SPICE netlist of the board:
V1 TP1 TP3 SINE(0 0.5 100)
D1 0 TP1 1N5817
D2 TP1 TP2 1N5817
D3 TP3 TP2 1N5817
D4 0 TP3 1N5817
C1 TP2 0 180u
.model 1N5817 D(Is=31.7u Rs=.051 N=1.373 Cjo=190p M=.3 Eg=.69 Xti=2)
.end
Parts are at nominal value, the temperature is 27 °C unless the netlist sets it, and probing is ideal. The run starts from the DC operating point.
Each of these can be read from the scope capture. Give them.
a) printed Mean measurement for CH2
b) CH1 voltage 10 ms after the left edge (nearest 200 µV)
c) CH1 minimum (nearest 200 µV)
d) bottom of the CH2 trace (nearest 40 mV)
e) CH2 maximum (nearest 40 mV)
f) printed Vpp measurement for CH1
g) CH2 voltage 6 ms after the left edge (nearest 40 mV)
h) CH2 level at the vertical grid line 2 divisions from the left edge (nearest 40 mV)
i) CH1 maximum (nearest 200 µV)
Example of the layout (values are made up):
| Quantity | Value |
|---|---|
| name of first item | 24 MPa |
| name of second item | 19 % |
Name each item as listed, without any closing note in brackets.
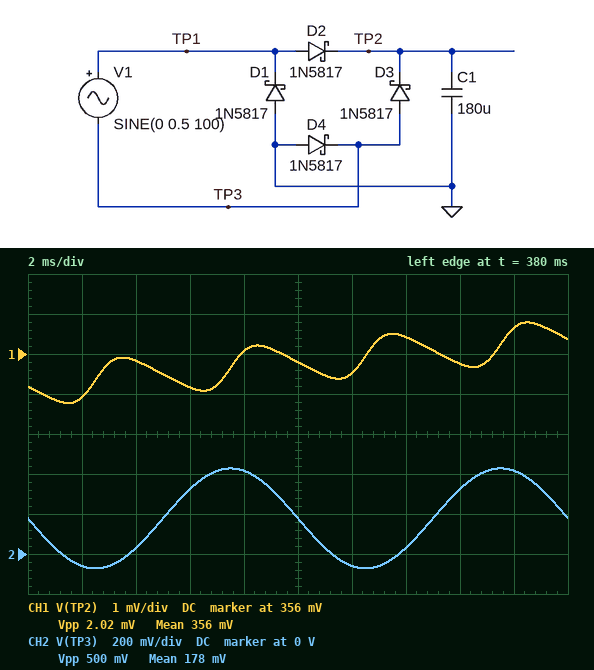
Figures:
| Quantity | Value |
|---|---|
| printed Mean measurement for CH2 | 178 mV |
| CH1 voltage 10 ms after the left edge | 355.8 mV |
| CH1 minimum | 354.8 mV |
| bottom of the CH2 trace | -80 mV |
| CH2 maximum | 440 mV |
| printed Vpp measurement for CH1 | 2.02 mV |
| CH2 voltage 6 ms after the left edge | 320 mV |
| CH2 level at the vertical grid line 2 divisions from the left edge | 40 mV |
| CH1 maximum | 356.8 mV |
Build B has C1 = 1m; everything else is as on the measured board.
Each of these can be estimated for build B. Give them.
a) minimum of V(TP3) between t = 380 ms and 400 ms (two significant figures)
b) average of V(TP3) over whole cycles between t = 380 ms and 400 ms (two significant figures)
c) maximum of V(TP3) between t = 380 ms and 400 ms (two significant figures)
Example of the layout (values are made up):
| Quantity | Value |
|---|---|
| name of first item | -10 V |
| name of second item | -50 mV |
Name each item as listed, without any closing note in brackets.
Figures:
| Quantity | Value |
|---|---|
| minimum of V(TP3) between t = 380 ms and 400 ms | -110 mV |
| average of V(TP3) over whole cycles between t = 380 ms and 400 ms | 140 mV |
| maximum of V(TP3) between t = 380 ms and 400 ms | 390 mV |
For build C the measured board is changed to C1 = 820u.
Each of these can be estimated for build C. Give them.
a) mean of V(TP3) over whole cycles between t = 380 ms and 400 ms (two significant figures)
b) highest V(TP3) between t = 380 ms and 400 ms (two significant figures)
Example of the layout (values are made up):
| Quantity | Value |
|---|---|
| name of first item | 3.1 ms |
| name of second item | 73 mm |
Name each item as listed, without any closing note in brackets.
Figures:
| Quantity | Value |
|---|---|
| mean of V(TP3) over whole cycles between t = 380 ms and 400 ms | 150 mV |
| highest V(TP3) between t = 380 ms and 400 ms | 400 mV |
